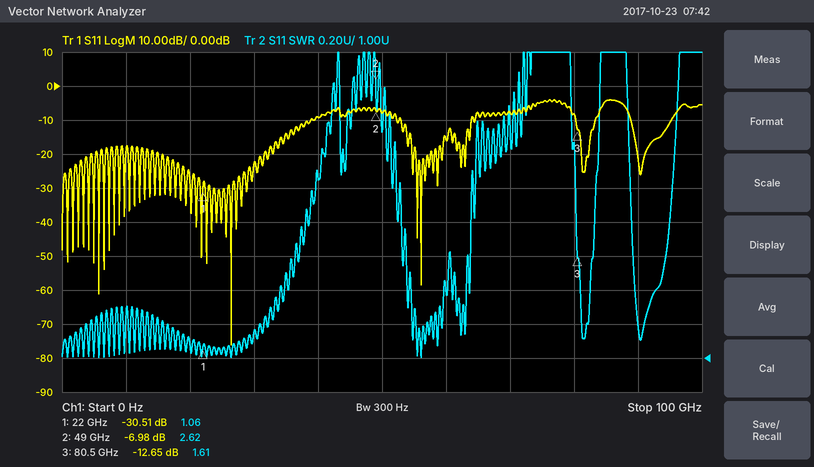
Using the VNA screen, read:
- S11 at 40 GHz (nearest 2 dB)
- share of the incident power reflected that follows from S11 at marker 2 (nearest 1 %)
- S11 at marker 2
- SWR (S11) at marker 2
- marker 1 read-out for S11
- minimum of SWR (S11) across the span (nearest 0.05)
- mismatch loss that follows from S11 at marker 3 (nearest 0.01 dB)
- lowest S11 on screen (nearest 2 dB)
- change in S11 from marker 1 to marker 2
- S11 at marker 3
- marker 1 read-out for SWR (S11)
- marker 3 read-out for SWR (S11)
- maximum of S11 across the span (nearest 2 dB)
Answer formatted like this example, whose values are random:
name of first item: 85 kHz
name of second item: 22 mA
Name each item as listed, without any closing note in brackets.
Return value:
S11 at 40 GHz: -10 dB
share of the incident power reflected that follows from S11 at marker 2: 20 %
S11 at marker 2: -6.98 dB
SWR (S11) at marker 2: 2.62
marker 1 read-out for S11: -30.51 dB
minimum of SWR (S11) across the span: 1.00
mismatch loss that follows from S11 at marker 3: 0.24 dB
lowest S11 on screen: -76 dB
change in S11 from marker 1 to marker 2: 23.53 dB
S11 at marker 3: -12.65 dB
marker 1 read-out for SWR: 1.06
marker 3 read-out for SWR: 1.61
maximum of S11 across the span: -4 dB
